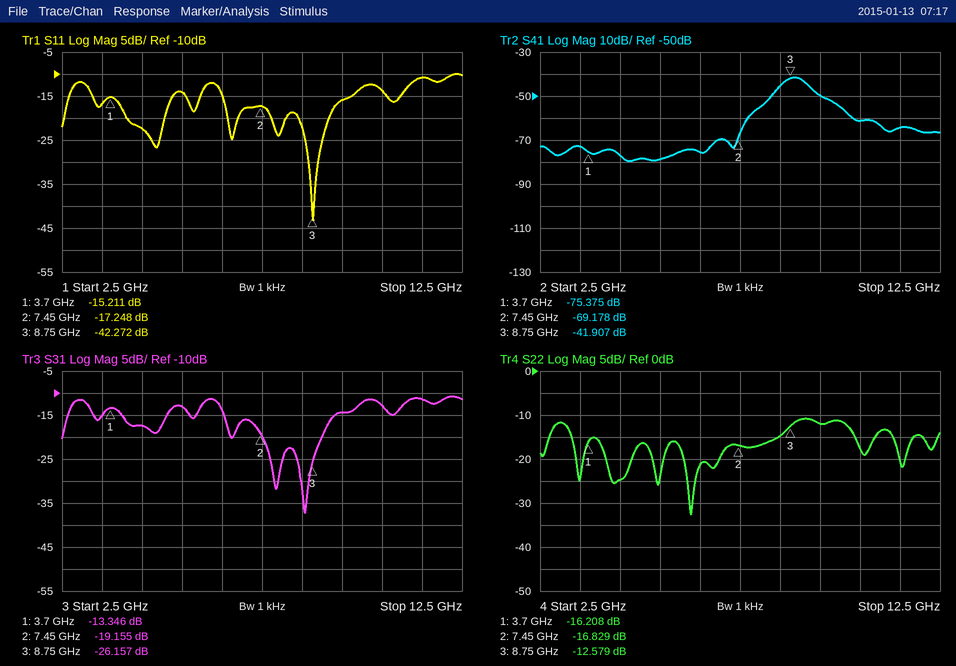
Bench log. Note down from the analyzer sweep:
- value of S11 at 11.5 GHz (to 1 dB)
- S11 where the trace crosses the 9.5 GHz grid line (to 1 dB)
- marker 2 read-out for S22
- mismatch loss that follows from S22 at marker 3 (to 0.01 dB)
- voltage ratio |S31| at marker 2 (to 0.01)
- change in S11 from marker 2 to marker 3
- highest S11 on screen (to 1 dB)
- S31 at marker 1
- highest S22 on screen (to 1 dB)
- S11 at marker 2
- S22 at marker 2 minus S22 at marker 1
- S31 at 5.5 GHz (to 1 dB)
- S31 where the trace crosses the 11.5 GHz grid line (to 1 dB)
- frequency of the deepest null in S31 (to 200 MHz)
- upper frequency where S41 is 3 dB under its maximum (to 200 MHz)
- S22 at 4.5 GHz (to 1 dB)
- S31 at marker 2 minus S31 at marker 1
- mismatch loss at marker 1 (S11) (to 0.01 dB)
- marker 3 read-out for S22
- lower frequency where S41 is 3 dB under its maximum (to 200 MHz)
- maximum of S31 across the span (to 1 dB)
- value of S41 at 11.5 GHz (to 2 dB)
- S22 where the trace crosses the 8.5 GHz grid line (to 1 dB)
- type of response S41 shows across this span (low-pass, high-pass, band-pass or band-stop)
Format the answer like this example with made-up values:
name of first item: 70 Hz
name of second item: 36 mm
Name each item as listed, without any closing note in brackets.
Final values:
value of S11 at 11.5 GHz: -11 dB
S11 where the trace crosses the 9.5 GHz grid line: -16 dB
marker 2 read-out for S22: -16.829 dB
mismatch loss that follows from S22 at marker 3: 0.25 dB
voltage ratio |S31| at marker 2: 0.11
change in S11 from marker 2 to marker 3: -25.024 dB
highest S11 on screen: -10 dB
S31 at marker 1: -13.346 dB
highest S22 on screen: -11 dB
S11 at marker 2: -17.248 dB
S22 at marker 2 minus S22 at marker 1: -0.621 dB
S31 at 5.5 GHz: -13 dB
S31 where the trace crosses the 11.5 GHz grid line: -11 dB
frequency of the deepest null in S31: 8.6 GHz
upper frequency where S41 is 3 dB under its maximum: 9.2 GHz
S22 at 4.5 GHz: -25 dB
S31 at marker 2 minus S31 at marker 1: -5.809 dB
mismatch loss at marker 1 (S11): 0.13 dB
marker 3 read-out for S22: -12.579 dB
lower frequency where S41 is 3 dB under its maximum: 8.6 GHz
maximum of S31 across the span: -11 dB
value of S41 at 11.5 GHz: -64 dB
S22 where the trace crosses the 8.5 GHz grid line: -15 dB
type of response S41 shows across this span: band-pass
